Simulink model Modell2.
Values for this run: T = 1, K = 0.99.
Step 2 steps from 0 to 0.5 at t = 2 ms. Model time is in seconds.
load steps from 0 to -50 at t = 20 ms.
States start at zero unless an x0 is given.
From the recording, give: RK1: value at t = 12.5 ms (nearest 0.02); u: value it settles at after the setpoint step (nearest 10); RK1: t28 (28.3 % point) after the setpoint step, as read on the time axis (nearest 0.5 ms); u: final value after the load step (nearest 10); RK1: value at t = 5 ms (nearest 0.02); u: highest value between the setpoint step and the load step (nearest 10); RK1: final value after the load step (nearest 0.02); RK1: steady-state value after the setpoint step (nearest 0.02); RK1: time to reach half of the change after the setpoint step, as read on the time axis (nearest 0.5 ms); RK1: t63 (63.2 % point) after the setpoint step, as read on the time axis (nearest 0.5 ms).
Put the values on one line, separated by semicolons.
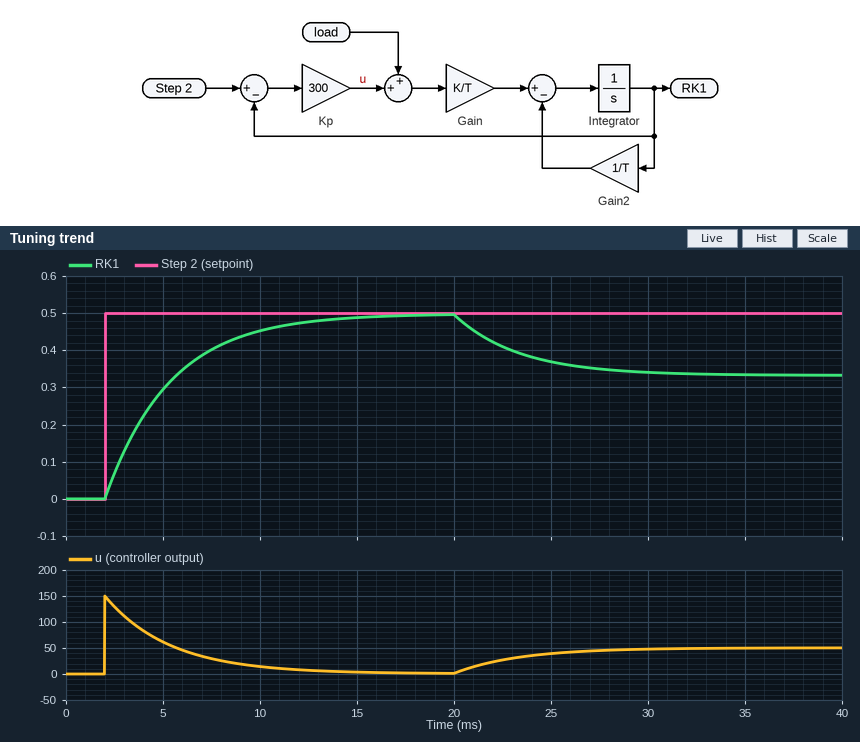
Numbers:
0.48; 0; 3.0 ms; 50; 0.30; 150; 0.34; 0.50; 4.5 ms; 5.5 ms
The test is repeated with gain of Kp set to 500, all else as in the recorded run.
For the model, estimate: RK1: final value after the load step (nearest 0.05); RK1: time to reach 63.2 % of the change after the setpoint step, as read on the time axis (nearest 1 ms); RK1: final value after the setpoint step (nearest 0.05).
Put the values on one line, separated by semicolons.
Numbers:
0.40; 4 ms; 0.50
